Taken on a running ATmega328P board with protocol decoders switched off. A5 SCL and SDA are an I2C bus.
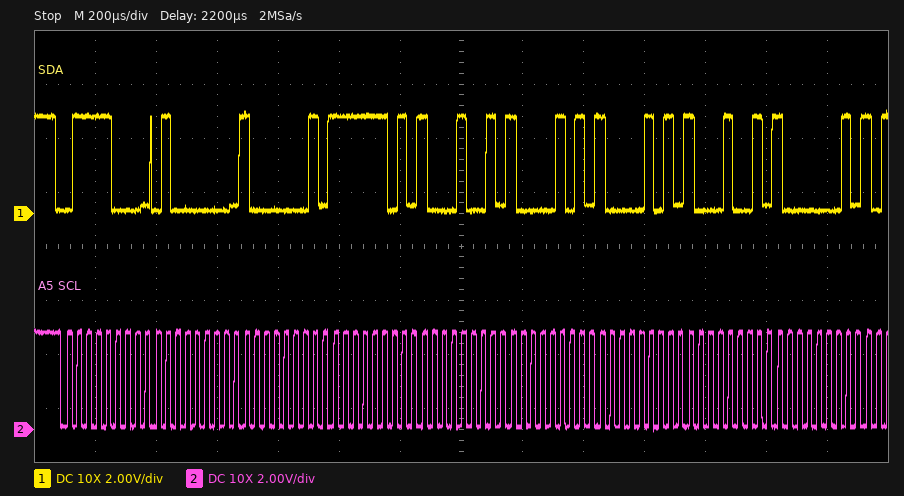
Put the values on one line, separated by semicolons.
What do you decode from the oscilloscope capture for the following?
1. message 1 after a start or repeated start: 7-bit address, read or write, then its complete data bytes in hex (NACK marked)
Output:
0x3C write: 40 81 FD 89 85 85 89 81
